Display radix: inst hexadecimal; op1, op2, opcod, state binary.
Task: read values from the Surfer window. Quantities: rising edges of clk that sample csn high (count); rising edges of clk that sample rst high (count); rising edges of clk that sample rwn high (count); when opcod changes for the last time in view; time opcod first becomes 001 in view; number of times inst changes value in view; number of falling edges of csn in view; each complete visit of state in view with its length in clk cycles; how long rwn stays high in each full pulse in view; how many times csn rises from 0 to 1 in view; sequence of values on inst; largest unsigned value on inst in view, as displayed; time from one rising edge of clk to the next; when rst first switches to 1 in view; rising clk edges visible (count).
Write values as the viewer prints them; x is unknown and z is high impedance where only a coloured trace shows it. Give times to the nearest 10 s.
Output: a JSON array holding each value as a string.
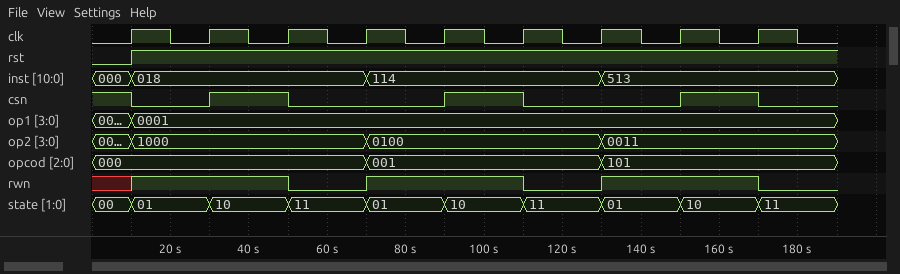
["4", "8", "6", "130 s", "70 s", "3", "4", "01: 1, 10: 1, 11: 1, 01: 1, 10: 1, 11: 1, 01: 1, 10: 1", "40 s, 40 s", "3", "000, 018, 114, 513", "513", "20 s", "10 s", "9"]
